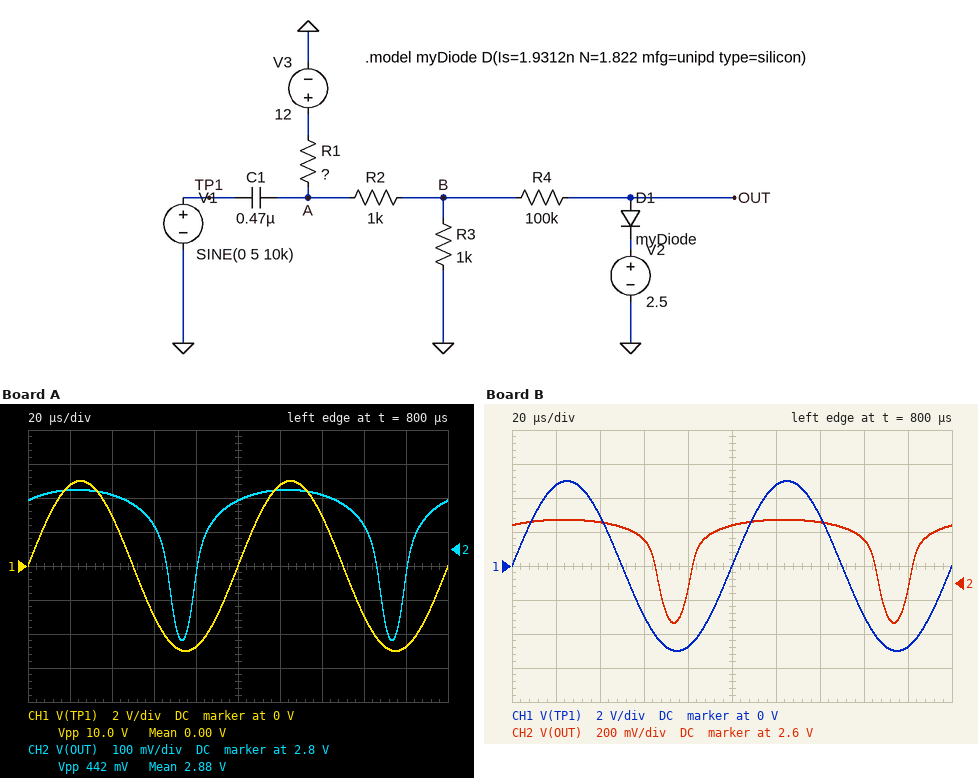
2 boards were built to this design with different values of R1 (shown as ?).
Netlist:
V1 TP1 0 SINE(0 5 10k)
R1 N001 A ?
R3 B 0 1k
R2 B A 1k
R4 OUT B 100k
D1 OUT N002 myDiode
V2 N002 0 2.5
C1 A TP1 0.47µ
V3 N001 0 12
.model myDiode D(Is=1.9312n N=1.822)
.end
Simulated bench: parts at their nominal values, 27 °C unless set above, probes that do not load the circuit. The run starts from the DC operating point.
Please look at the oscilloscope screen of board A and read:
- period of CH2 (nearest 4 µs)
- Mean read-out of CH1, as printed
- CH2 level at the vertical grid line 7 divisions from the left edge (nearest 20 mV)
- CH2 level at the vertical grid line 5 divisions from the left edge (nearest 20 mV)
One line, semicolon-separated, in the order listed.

100 µs; 0.00 V; 2.96 V; 2.94 V
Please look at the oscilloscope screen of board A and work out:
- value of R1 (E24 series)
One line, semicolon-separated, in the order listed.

390 Ω
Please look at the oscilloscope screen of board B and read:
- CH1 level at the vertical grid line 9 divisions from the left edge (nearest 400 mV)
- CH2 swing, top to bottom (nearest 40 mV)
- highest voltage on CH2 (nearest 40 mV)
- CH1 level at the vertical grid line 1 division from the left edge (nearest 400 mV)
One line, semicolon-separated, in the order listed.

-4.8 V; 600 mV; 2.96 V; 4.8 V
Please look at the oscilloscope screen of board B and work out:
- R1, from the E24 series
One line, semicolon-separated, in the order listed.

470 Ω
